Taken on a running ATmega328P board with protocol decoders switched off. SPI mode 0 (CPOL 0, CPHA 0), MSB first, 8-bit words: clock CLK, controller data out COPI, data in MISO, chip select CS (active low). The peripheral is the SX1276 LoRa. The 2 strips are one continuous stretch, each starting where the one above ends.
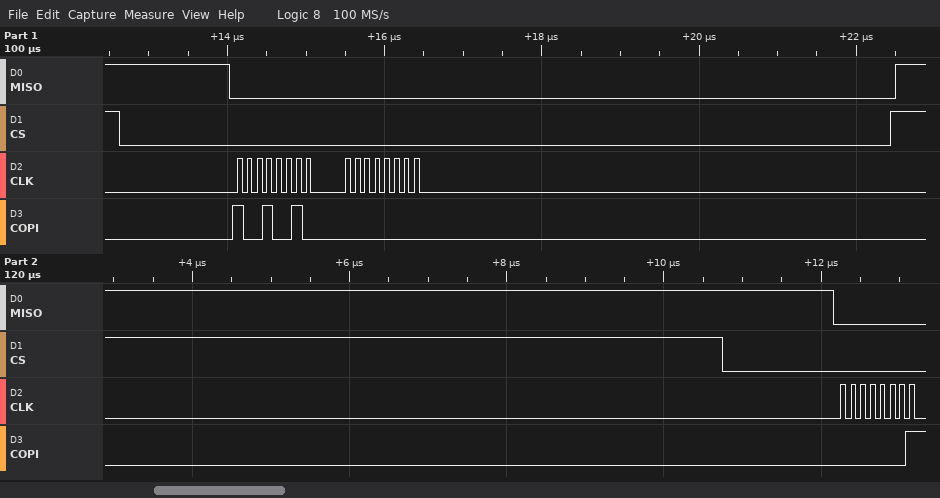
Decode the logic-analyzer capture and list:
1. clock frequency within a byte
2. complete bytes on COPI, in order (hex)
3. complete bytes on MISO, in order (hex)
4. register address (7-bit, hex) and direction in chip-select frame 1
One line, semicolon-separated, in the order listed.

8 MHz; 0x92 0x00 0x01; 0x00 0x00 0x00; 0x12 write
